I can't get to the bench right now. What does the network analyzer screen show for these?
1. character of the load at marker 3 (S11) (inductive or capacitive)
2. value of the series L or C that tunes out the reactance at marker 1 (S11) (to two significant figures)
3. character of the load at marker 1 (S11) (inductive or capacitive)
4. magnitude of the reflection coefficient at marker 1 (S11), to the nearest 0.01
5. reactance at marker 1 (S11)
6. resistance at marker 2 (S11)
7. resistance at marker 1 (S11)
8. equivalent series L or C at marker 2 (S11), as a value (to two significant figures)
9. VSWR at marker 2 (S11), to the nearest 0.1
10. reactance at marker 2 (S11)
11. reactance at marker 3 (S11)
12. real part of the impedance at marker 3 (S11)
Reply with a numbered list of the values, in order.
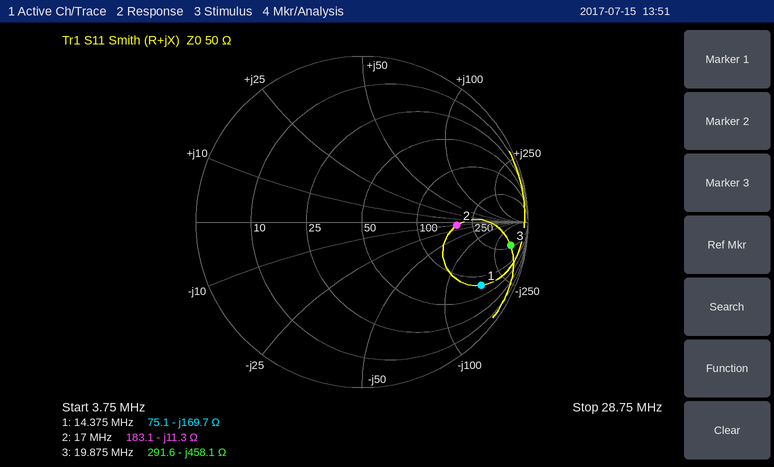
1. capacitive
2. 1.9 µH
3. capacitive
4. 0.81
5. -169.7 Ω
6. 183.1 Ω
7. 75.1 Ω
8. 830 pF
9. 3.7
10. -11.3 Ω
11. -458.1 Ω
12. 291.6 Ω
